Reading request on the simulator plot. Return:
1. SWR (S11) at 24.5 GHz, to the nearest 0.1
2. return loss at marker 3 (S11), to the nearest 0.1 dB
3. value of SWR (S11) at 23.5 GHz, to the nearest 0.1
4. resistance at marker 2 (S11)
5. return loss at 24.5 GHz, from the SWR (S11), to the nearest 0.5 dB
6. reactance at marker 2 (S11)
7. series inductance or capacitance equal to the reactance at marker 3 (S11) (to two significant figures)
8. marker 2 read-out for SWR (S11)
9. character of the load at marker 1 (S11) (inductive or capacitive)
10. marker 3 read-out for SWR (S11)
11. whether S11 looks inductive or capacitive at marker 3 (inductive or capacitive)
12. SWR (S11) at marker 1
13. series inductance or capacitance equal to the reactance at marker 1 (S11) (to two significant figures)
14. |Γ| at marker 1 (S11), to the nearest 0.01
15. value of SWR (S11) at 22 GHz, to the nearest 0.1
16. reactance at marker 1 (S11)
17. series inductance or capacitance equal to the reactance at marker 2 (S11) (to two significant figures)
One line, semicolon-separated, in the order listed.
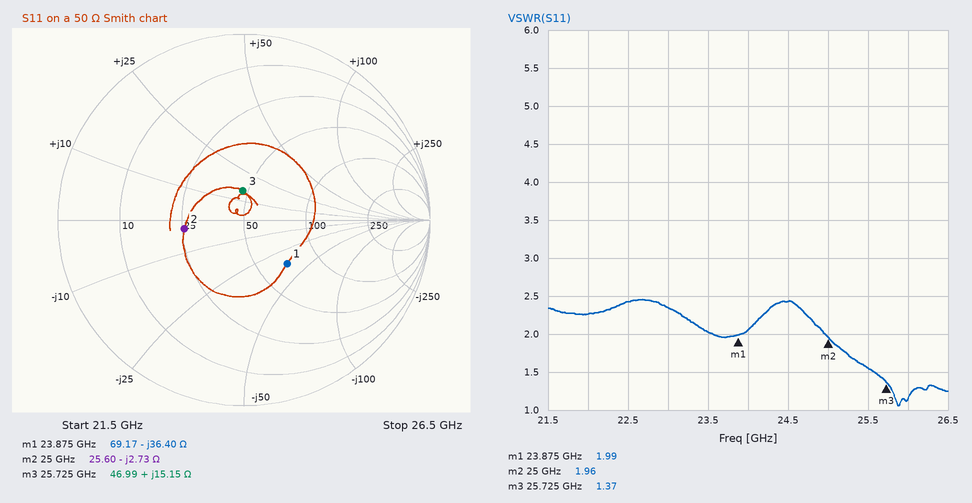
2.4; 16.1 dB; 2.0; 25.60 Ω; 7.5 dB; -2.73 Ω; 94 pH; 1.96; capacitive; 1.37; inductive; 1.99; 180 fF; 0.33; 2.3; -36.40 Ω; 2.3 pF
